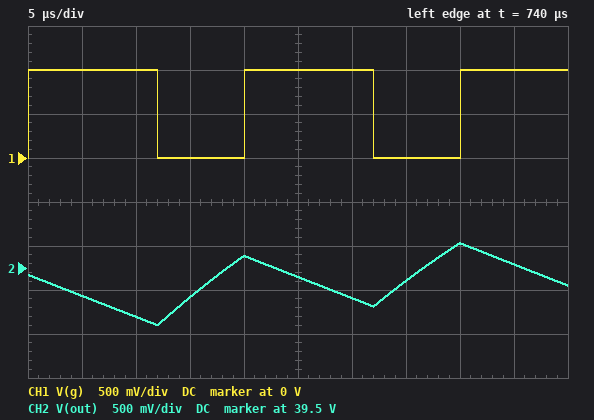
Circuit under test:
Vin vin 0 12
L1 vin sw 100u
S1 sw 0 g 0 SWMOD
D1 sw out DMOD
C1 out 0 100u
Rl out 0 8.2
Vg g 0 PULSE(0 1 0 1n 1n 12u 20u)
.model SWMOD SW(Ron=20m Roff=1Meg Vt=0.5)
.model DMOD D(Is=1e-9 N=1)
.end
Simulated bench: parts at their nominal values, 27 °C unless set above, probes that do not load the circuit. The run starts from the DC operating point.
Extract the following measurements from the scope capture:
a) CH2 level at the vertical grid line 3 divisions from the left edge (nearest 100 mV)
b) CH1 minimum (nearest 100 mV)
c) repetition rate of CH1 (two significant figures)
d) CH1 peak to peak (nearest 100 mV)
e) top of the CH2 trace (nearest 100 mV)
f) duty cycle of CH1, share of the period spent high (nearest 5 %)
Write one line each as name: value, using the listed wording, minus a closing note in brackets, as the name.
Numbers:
CH2 level at the vertical grid line 3 divisions from the left edge: 39.2 V
CH1 minimum: 0 V
repetition rate of CH1: 50 kHz
CH1 peak to peak: 1.0 V
top of the CH2 trace: 39.8 V
duty cycle of CH1, share of the period spent high: 60 %
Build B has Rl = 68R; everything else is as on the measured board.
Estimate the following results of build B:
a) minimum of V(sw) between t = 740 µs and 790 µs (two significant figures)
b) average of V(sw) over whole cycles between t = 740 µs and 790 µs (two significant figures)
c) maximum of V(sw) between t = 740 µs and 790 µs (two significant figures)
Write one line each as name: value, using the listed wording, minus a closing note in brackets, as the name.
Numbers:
minimum of V(sw) between t = 740 µs and 790 µs: 18 mV
average of V(sw) over whole cycles between t = 740 µs and 790 µs: 18 V
maximum of V(sw) between t = 740 µs and 790 µs: 46 V
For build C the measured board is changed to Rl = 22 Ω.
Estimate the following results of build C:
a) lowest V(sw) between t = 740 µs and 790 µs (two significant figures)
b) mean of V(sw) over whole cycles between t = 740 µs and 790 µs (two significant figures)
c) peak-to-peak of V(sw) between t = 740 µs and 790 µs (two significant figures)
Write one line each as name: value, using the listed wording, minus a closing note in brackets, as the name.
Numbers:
lowest V(sw) between t = 740 µs and 790 µs: 93 mV
mean of V(sw) over whole cycles between t = 740 µs and 790 µs: 18 V
peak-to-peak of V(sw) between t = 740 µs and 790 µs: 44 V
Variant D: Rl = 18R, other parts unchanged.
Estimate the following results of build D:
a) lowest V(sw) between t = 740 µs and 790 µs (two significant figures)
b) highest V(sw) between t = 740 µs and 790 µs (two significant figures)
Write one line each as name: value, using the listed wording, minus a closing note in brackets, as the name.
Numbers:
lowest V(sw) between t = 740 µs and 790 µs: 120 mV
highest V(sw) between t = 740 µs and 790 µs: 44 V
